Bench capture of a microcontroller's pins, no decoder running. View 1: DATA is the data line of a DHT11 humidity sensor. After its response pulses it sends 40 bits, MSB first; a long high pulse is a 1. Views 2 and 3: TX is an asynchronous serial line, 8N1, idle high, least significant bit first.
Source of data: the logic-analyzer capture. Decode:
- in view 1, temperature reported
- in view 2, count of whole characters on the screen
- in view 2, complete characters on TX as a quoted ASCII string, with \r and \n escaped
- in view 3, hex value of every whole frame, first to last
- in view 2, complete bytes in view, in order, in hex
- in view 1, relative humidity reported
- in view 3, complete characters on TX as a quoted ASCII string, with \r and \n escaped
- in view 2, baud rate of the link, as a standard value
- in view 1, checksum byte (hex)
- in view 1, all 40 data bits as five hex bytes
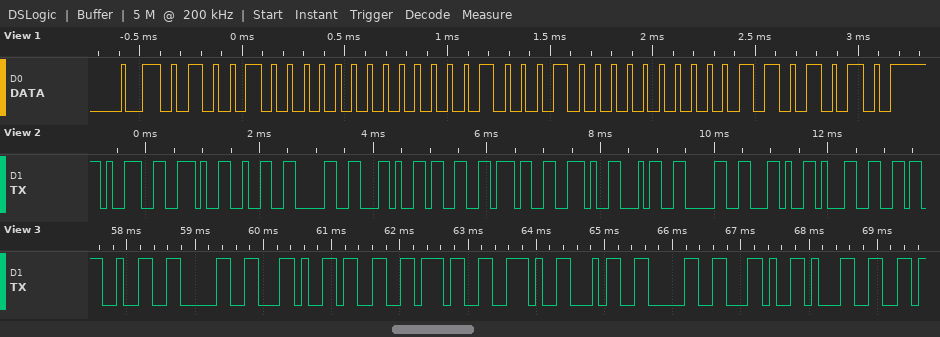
34.0 °C
12
"9.20,37.40,1"
32 30 2C 33 37 2E 34 30 2C 31
0x39 0x2E 0x32 0x30 0x2C 0x33 0x37 0x2E 0x34 0x30 0x2C 0x31
72 %
"20,37.40,1"
9600 baud
0x6A
48 00 22 00 6A
